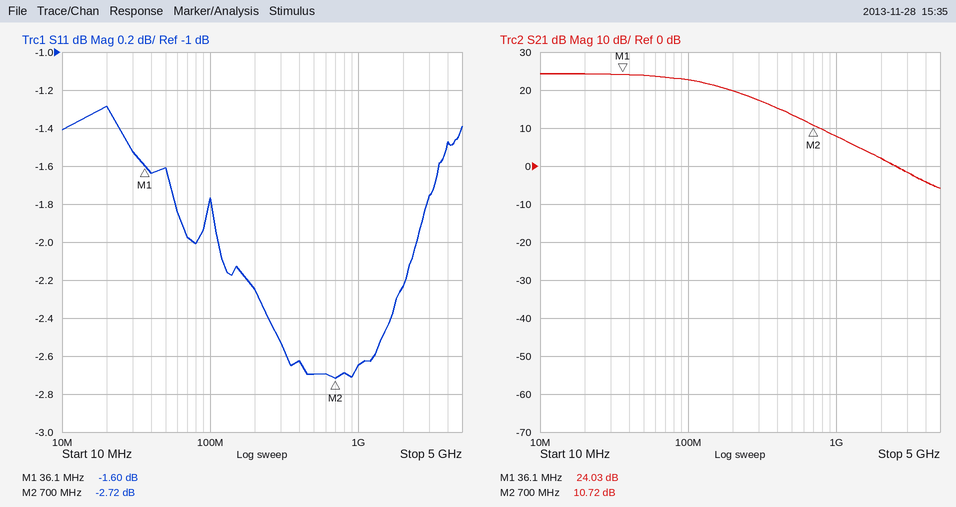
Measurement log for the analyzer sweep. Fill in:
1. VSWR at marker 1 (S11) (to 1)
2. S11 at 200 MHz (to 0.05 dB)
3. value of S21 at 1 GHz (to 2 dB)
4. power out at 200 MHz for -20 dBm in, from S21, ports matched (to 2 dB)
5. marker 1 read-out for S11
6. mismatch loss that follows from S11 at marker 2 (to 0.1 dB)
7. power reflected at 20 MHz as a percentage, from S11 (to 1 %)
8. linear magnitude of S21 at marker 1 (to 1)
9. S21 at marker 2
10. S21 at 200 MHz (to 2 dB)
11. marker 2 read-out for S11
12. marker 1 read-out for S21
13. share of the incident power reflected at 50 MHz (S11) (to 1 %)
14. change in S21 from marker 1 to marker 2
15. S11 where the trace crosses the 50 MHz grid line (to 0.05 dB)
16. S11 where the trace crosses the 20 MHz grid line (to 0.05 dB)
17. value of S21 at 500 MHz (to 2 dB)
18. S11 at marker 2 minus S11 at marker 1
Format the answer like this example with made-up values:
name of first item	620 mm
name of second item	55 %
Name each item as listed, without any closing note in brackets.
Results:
VSWR at marker 1 (S11)	11
S11 at 200 MHz	-2.25 dB
value of S21 at 1 GHz	8 dB
power out at 200 MHz for -20 dBm in, from S21, ports matched	0 dBm
marker 1 read-out for S11	-1.60 dB
mismatch loss that follows from S11 at marker 2	3.3 dB
power reflected at 20 MHz as a percentage, from S11	74 %
linear magnitude of S21 at marker 1	16
S21 at marker 2	10.72 dB
S21 at 200 MHz	20 dB
marker 2 read-out for S11	-2.72 dB
marker 1 read-out for S21	24.03 dB
share of the incident power reflected at 50 MHz (S11)	69 %
change in S21 from marker 1 to marker 2	-13.31 dB
S11 where the trace crosses the 50 MHz grid line	-1.60 dB
S11 where the trace crosses the 20 MHz grid line	-1.30 dB
value of S21 at 500 MHz	14 dB
S11 at marker 2 minus S11 at marker 1	-1.12 dB
